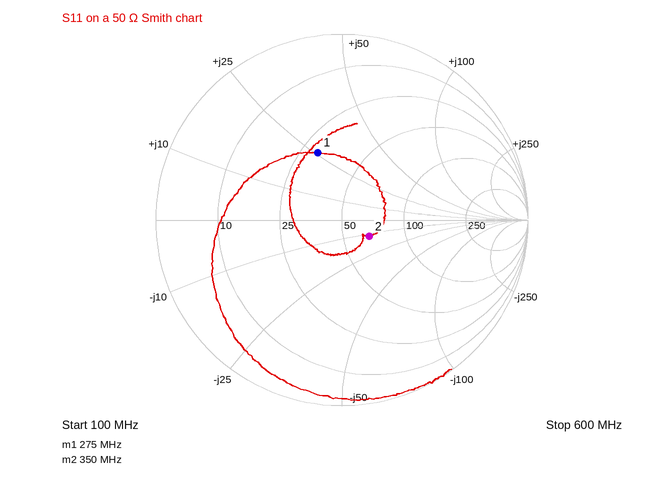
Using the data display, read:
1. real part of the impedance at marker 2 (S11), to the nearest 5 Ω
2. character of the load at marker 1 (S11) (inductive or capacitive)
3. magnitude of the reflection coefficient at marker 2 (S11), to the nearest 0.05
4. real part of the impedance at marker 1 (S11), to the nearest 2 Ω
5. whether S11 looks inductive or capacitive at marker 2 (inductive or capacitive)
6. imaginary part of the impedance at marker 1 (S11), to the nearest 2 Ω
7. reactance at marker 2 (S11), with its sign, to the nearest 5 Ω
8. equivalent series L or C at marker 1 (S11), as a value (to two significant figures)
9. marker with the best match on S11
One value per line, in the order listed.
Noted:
65 Ω
inductive
0.15
30 Ω
capacitive
+26 Ω
-10 Ω
15 nH
marker 2
